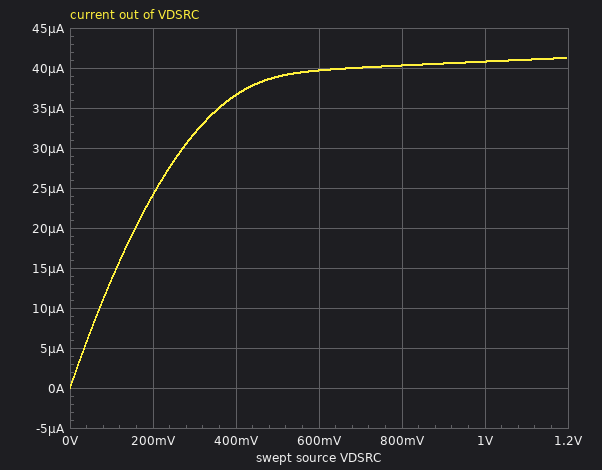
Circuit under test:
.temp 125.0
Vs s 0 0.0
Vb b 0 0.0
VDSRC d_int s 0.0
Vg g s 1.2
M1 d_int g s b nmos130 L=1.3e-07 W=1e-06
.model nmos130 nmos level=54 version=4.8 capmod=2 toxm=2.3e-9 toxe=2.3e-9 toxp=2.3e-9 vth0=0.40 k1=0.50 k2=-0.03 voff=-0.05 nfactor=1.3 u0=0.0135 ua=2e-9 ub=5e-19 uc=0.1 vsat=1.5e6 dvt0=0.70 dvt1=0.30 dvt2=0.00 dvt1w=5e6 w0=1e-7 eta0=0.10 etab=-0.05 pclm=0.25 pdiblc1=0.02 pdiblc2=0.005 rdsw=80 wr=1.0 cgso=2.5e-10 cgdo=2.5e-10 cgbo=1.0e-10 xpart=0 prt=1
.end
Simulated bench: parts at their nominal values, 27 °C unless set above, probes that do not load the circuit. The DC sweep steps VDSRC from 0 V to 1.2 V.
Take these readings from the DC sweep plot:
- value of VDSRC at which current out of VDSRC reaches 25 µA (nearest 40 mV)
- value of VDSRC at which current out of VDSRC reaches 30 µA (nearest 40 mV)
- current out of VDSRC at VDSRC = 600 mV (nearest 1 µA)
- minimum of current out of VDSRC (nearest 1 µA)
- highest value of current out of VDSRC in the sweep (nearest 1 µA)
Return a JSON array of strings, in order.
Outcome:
["200 mV", "280 mV", "40 µA", "0 A", "41 µA"]
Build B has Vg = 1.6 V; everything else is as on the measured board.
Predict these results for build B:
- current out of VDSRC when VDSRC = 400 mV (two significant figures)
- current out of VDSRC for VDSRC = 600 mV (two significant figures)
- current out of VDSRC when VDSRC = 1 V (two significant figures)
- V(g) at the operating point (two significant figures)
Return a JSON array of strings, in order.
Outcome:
["74 µA", "95 µA", "110 µA", "1.6 V"]
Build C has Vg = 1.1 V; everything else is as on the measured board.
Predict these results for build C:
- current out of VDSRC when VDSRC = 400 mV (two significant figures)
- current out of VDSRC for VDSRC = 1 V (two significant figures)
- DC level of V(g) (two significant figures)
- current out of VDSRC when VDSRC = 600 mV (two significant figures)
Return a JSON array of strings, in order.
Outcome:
["25 µA", "27 µA", "1.1 V", "26 µA"]
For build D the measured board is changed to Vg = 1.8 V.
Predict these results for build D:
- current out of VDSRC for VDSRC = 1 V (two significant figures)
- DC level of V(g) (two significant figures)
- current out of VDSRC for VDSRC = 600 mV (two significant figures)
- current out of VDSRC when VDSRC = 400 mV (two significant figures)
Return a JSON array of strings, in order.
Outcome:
["150 µA", "1.8 V", "120 µA", "90 µA"]
